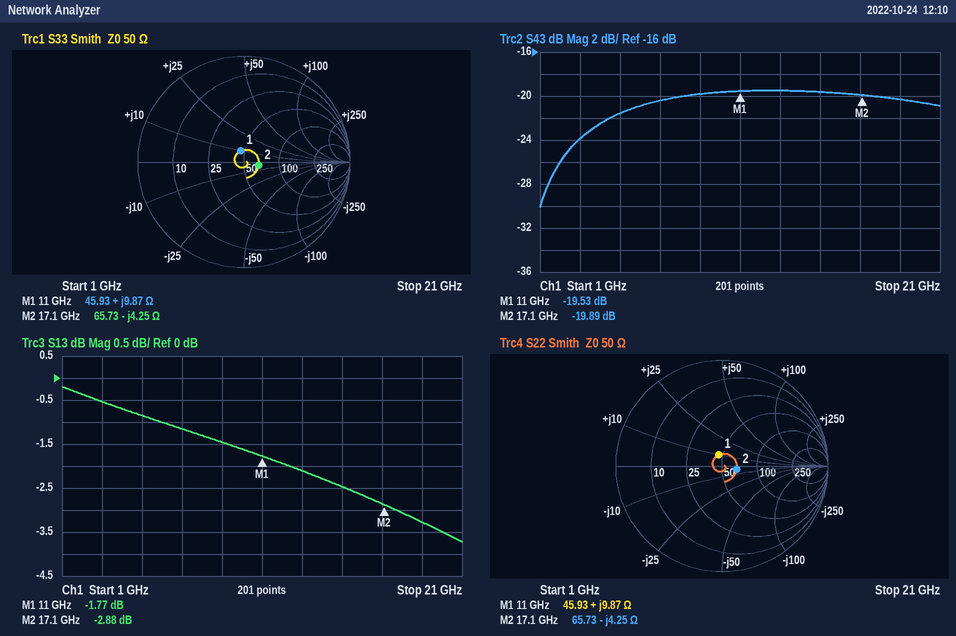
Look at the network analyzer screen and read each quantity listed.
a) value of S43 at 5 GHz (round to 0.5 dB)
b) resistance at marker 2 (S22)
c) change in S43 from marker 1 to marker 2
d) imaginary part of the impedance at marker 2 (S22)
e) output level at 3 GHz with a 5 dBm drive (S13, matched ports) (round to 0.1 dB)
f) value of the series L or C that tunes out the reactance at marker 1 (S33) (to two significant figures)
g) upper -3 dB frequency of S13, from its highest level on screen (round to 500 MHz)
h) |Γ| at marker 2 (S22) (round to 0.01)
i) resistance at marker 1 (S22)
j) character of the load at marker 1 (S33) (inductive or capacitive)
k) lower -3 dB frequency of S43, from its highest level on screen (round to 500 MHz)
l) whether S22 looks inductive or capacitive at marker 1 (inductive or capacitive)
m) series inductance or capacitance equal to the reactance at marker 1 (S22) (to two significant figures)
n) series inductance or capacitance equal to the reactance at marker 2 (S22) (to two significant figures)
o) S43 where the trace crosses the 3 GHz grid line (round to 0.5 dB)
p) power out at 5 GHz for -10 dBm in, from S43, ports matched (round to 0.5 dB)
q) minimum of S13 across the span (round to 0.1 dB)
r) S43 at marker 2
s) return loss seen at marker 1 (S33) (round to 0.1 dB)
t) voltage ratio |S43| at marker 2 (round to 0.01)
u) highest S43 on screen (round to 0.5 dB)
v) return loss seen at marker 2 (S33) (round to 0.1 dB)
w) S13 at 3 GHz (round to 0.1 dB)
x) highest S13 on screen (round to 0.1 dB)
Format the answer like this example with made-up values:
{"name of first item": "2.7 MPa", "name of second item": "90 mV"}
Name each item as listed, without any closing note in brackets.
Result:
{"value of S43 at 5 GHz": "-21.5 dB", "resistance at marker 2": "65.73 Ω", "change in S43 from marker 1 to marker 2": "-0.36 dB", "imaginary part of the impedance at marker 2": "-4.25 Ω", "output level at 3 GHz with a 5 dBm drive (S13, matched ports)": "4.5 dBm", "value of the series L or C that tunes out the reactance at marker 1 (S33)": "1.5 pF", "upper -3 dB frequency of S13, from its highest level on screen": "18.5 GHz", "|Γ| at marker 2 (S22)": "0.14", "resistance at marker 1": "45.93 Ω", "character of the load at marker 1 (S33)": "inductive", "lower -3 dB frequency of S43, from its highest level on screen": "4.0 GHz", "whether S22 looks inductive or capacitive at marker 1": "inductive", "series inductance or capacitance equal to the reactance at marker 1 (S22)": "140 pH", "series inductance or capacitance equal to the reactance at marker 2 (S22)": "2.2 pF", "S43 where the trace crosses the 3 GHz grid line": "-24.0 dB", "power out at 5 GHz for -10 dBm in, from S43, ports matched": "-31.5 dBm", "minimum of S13 across the span": "-3.7 dB", "S43 at marker 2": "-19.89 dB", "return loss seen at marker 1 (S33)": "19.1 dB", "voltage ratio |S43| at marker 2": "0.10", "highest S43 on screen": "-19.5 dB", "return loss seen at marker 2 (S33)": "17.0 dB", "S13 at 3 GHz": "-0.5 dB", "highest S13 on screen": "-0.2 dB"}
